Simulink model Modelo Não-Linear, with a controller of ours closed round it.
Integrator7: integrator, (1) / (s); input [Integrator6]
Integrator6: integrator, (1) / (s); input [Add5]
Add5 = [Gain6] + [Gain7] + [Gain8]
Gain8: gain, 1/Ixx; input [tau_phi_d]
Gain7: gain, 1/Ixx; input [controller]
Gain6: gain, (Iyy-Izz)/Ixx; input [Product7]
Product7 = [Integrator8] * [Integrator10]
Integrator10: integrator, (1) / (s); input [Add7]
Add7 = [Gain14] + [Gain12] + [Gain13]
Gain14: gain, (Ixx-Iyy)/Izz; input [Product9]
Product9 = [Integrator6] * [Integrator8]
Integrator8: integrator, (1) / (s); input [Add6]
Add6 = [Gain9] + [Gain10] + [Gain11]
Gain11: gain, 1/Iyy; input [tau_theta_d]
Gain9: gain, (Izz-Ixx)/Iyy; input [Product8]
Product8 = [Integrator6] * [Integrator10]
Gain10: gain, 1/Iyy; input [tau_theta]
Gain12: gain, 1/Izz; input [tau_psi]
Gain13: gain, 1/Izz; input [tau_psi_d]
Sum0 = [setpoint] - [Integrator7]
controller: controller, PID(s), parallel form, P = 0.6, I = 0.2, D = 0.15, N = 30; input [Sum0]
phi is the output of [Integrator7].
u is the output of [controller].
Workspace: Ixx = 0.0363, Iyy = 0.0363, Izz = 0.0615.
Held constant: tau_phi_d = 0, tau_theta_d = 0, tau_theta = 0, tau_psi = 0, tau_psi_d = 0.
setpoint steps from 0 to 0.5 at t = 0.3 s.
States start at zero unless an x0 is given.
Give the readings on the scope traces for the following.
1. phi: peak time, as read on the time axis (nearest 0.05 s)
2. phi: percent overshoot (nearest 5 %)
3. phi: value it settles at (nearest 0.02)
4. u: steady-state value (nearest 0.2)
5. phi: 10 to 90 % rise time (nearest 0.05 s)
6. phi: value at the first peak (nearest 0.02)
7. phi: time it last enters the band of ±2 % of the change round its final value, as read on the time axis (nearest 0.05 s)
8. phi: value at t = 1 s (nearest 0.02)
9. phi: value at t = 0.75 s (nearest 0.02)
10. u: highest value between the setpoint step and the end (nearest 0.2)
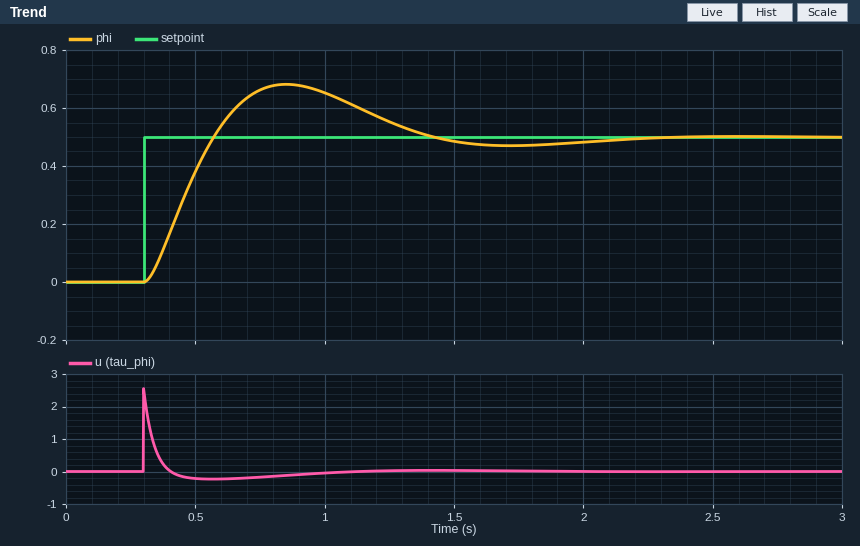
0.85 s
35 %
0.50
0.0
0.20 s
0.68
2.15 s
0.66
0.66
2.6
